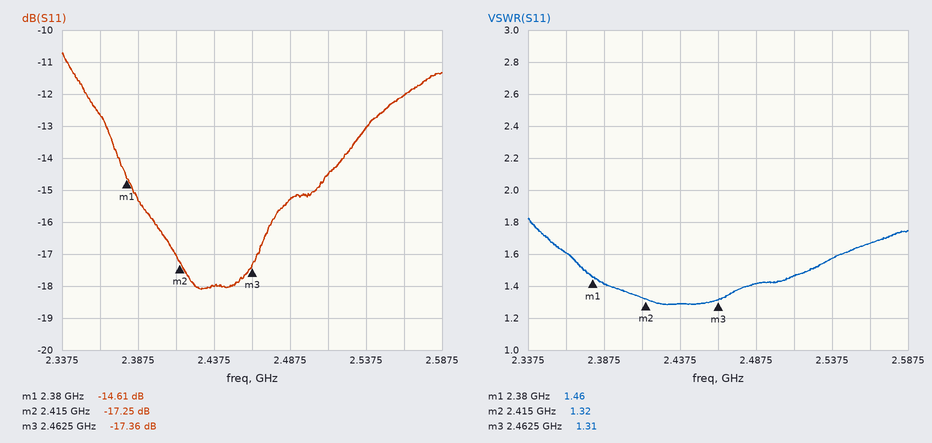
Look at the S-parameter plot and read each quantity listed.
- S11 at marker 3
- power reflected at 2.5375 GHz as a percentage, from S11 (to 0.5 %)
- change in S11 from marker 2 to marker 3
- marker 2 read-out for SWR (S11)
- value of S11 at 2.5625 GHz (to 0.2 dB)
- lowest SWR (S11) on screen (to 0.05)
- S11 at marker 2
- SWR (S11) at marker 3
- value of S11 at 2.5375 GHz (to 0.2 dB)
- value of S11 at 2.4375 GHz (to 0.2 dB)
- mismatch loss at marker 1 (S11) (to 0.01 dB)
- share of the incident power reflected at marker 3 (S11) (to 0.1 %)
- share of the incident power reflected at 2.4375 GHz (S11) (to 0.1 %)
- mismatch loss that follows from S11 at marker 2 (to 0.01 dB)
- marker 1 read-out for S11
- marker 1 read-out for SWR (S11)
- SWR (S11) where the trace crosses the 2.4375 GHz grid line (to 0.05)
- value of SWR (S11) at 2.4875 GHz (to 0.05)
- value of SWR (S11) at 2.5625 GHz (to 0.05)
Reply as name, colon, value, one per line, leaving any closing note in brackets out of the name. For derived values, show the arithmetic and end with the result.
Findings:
S11 at marker 3: -17.36 dB
power reflected at 2.5375 GHz as a percentage, from S11: 10^(-13/10) ≈ 5.0 %
change in S11 from marker 2 to marker 3: -17.36 − (-17.25) = -0.11 dB
marker 2 read-out for SWR: 1.32
value of S11 at 2.5625 GHz: -12.0 dB
lowest SWR (S11) on screen: 1.30
S11 at marker 2: -17.25 dB
SWR (S11) at marker 3: 1.31
value of S11 at 2.5375 GHz: -13.0 dB
value of S11 at 2.4375 GHz: -18.0 dB
mismatch loss at marker 1 (S11): −10 log10(1 − 10^(-14.61/10)) ≈ 0.15 dB
share of the incident power reflected at marker 3 (S11): 10^(-17.36/10) ≈ 1.8 %
share of the incident power reflected at 2.4375 GHz (S11): 10^(-18/10) ≈ 1.6 %
mismatch loss that follows from S11 at marker 2: −10 log10(1 − 10^(-17.25/10)) ≈ 0.08 dB
marker 1 read-out for S11: -14.61 dB
marker 1 read-out for SWR: 1.46
SWR (S11) where the trace crosses the 2.4375 GHz grid line: 1.30
value of SWR (S11) at 2.4875 GHz: 1.40
value of SWR (S11) at 2.5625 GHz: 1.65
